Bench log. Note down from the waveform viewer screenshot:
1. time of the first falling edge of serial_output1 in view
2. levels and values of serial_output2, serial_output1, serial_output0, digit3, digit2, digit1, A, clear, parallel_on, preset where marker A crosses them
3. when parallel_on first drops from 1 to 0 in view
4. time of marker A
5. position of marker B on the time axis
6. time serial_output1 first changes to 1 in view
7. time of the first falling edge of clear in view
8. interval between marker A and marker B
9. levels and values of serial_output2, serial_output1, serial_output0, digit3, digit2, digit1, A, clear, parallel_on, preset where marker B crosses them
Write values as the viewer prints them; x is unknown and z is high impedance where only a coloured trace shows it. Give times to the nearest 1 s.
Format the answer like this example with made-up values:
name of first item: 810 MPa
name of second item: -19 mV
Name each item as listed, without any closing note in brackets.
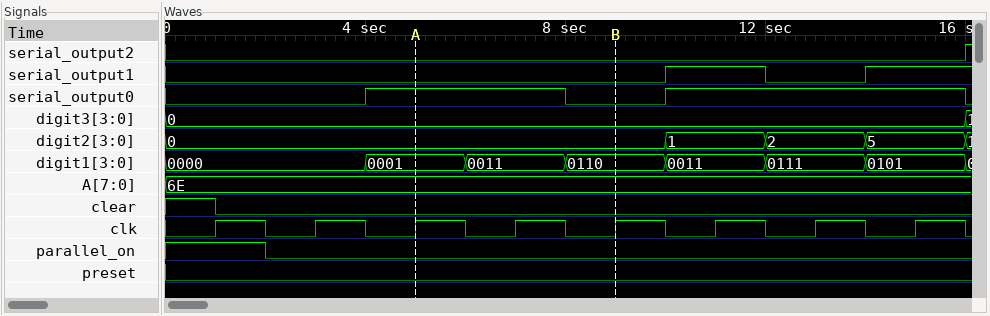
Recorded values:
time of the first falling edge of serial_output1 in view: 12 s
levels and values of serial_output2, serial_output1, serial_output0, digit3, digit2, digit1, A, clear, parallel_on, preset where marker A crosses them: serial_output2=0, serial_output1=0, serial_output0=1, digit3=0, digit2=0, digit1=0001, A=6E, clear=0, parallel_on=0, preset=0
when parallel_on first drops from 1 to 0 in view: 2 s
time of marker A: 5 s
position of marker B on the time axis: 9 s
time serial_output1 first changes to 1 in view: 10 s
time of the first falling edge of clear in view: 1 s
interval between marker A and marker B: 4 s
levels and values of serial_output2, serial_output1, serial_output0, digit3, digit2, digit1, A, clear, parallel_on, preset where marker B crosses them: serial_output2=0, serial_output1=0, serial_output0=0, digit3=0, digit2=0, digit1=0110, A=6E, clear=0, parallel_on=0, preset=0
